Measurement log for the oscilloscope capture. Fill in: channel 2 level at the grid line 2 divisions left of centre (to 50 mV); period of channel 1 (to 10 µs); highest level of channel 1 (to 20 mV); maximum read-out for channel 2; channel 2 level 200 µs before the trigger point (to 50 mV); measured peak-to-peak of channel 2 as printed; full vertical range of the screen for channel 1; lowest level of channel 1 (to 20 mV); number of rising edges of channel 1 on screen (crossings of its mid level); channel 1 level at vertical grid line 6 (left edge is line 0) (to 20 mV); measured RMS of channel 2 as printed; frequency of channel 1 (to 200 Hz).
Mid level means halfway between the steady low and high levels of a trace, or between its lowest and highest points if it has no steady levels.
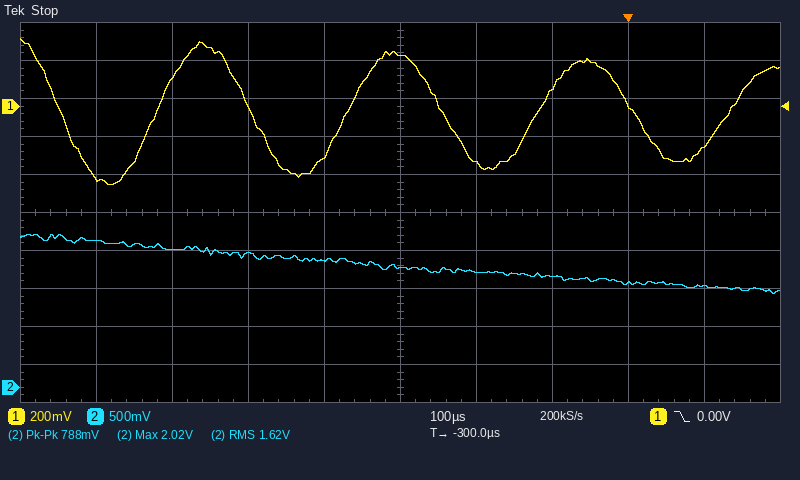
1.75 V
250 µs
360 mV
2.02 V
1.50 V
788 mV
2 V
-420 mV
4
-300 mV
1.62 V
4.0 kHz
